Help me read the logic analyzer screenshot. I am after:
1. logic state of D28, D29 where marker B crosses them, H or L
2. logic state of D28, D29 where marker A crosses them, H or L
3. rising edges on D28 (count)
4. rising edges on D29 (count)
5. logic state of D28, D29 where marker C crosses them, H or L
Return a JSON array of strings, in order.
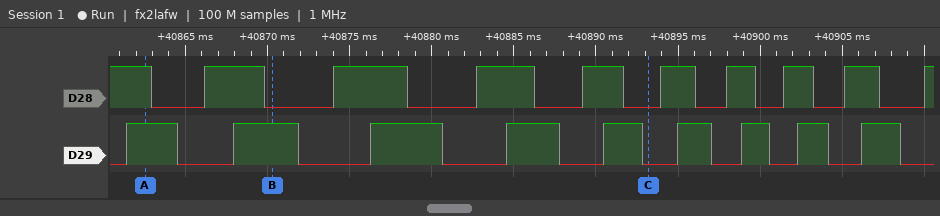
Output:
["D28=L, D29=H", "D28=H, D29=H", "9", "9", "D28=L, D29=L"]
